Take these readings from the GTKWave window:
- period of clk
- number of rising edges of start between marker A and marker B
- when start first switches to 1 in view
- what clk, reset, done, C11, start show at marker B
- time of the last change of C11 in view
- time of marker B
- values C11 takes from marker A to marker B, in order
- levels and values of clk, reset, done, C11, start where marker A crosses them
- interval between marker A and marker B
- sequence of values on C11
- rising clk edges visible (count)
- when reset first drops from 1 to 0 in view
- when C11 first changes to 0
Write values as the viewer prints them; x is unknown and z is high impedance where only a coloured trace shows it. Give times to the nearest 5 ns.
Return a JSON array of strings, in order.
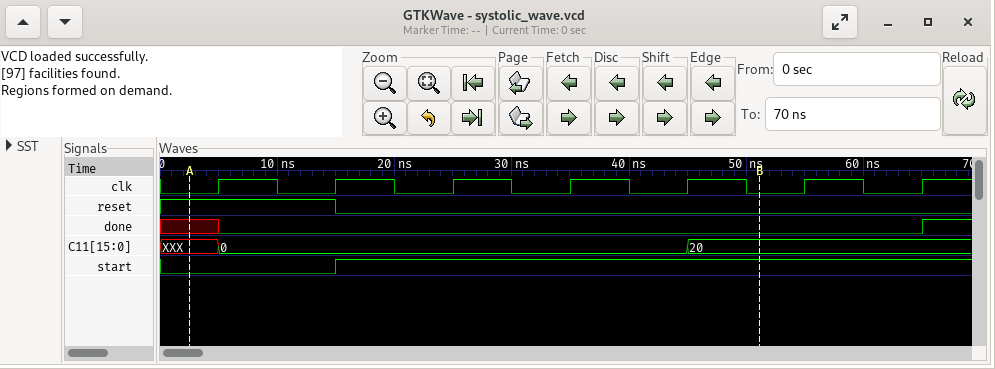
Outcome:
["10 ns", "1", "15 ns", "clk=0, reset=0, done=0, C11=20, start=1", "45 ns", "50 ns", "XXX, 0, 20", "clk=0, reset=1, done=x, C11=XXX, start=0", "50 ns", "XXX, 0, 20", "7", "15 ns", "5 ns"]
